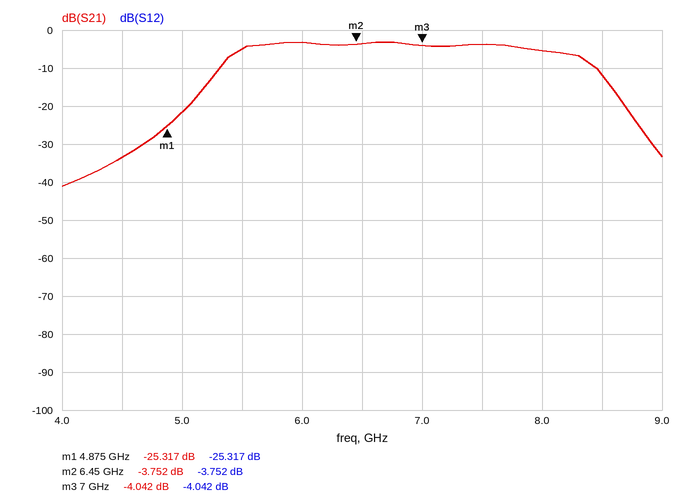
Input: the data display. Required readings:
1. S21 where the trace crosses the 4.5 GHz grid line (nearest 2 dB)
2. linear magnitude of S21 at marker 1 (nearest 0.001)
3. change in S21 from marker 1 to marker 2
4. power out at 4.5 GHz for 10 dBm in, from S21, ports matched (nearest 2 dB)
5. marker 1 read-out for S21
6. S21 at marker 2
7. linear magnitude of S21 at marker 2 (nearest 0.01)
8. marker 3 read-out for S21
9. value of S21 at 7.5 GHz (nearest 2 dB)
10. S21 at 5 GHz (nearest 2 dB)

-34 dB
0.054
21.565 dB
-24 dBm
-25.317 dB
-3.752 dB
0.65
-4.042 dB
-4 dB
-22 dB
